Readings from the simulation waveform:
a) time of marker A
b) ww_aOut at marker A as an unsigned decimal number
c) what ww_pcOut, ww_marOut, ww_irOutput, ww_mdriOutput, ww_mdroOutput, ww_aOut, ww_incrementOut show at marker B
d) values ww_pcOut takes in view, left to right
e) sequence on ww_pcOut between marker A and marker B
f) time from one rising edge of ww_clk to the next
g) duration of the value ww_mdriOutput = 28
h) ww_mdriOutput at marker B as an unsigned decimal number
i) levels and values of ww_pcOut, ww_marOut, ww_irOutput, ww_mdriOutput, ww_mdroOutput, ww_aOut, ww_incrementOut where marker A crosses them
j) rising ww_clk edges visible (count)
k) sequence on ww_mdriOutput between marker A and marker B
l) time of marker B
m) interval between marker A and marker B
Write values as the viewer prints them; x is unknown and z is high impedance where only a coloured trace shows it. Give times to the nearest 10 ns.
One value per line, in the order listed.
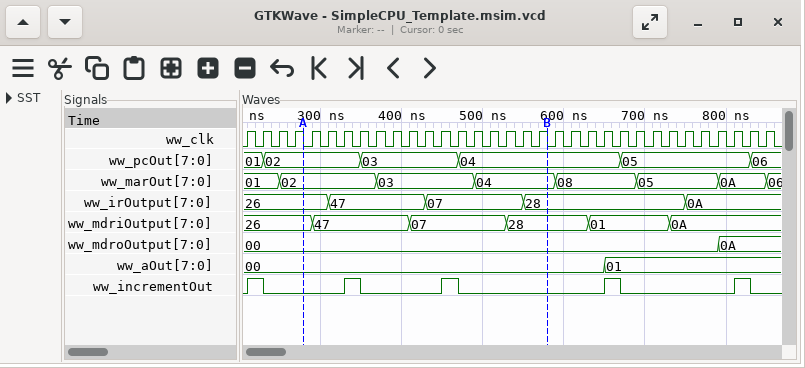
280 ns
0
ww_pcOut=04, ww_marOut=04, ww_irOutput=28, ww_mdriOutput=28, ww_mdroOutput=00, ww_aOut=00, ww_incrementOut=0
01, 02, 03, 04, 05, 06
02, 03, 04
20 ns
100 ns
40
ww_pcOut=02, ww_marOut=02, ww_irOutput=26, ww_mdriOutput=26, ww_mdroOutput=00, ww_aOut=00, ww_incrementOut=0
33
26, 47, 07, 28
580 ns
300 ns
